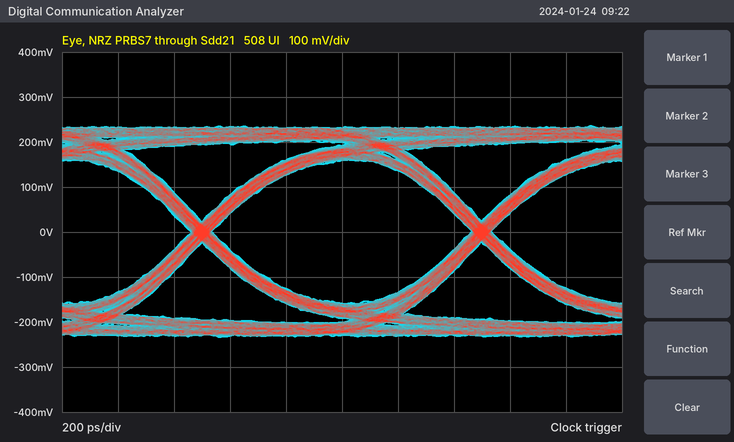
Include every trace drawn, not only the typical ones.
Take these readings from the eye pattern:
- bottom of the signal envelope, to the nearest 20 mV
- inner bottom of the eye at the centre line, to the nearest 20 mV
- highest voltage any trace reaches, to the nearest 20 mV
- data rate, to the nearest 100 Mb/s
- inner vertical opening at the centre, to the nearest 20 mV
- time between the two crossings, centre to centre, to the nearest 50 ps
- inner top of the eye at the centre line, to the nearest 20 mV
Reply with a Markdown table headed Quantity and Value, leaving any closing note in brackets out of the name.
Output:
| Quantity | Value |
|---|---|
| bottom of the signal envelope, to the nearest 20 mV | -240 mV |
| inner bottom of the eye at the centre line, to the nearest 20 mV | -160 mV |
| highest voltage any trace reaches, to the nearest 20 mV | 240 mV |
| data rate, to the nearest 100 Mb/s | 1.0 Gb/s |
| inner vertical opening at the centre, to the nearest 20 mV | 320 mV |
| time between the two crossings, centre to centre, to the nearest 50 ps | 1.00 ns |
| inner top of the eye at the centre line, to the nearest 20 mV | 160 mV |
